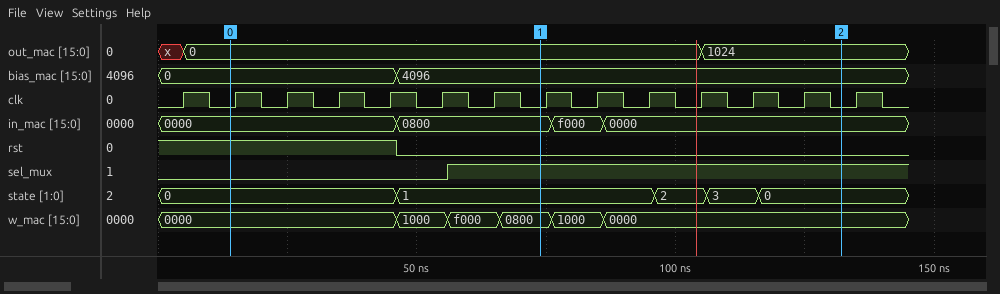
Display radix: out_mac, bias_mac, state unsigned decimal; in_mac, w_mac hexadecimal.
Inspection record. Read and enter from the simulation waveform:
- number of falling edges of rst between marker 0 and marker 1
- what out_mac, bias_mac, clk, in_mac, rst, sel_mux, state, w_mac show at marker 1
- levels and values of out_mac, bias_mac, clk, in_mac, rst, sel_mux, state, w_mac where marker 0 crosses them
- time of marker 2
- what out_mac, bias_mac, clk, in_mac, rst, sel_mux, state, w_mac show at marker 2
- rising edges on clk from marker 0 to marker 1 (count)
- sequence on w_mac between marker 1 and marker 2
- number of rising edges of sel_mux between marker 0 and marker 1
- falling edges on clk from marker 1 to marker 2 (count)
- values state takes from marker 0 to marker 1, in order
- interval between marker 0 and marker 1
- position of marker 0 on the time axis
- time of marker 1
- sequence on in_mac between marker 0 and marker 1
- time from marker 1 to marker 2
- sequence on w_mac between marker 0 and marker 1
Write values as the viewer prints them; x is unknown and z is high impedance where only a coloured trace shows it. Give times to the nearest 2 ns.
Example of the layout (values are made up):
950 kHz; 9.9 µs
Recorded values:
1; out_mac=0, bias_mac=4096, clk=0, in_mac=0800, rst=0, sel_mux=1, state=1, w_mac=0800; out_mac=0, bias_mac=0, clk=0, in_mac=0000, rst=1, sel_mux=0, state=0, w_mac=0000; 132 ns; out_mac=1024, bias_mac=4096, clk=0, in_mac=0000, rst=0, sel_mux=1, state=0, w_mac=0000; 6; 0800, 1000, 0000; 1; 6; 0, 1; 60 ns; 14 ns; 74 ns; 0000, 0800; 58 ns; 0000, 1000, f000, 0800
